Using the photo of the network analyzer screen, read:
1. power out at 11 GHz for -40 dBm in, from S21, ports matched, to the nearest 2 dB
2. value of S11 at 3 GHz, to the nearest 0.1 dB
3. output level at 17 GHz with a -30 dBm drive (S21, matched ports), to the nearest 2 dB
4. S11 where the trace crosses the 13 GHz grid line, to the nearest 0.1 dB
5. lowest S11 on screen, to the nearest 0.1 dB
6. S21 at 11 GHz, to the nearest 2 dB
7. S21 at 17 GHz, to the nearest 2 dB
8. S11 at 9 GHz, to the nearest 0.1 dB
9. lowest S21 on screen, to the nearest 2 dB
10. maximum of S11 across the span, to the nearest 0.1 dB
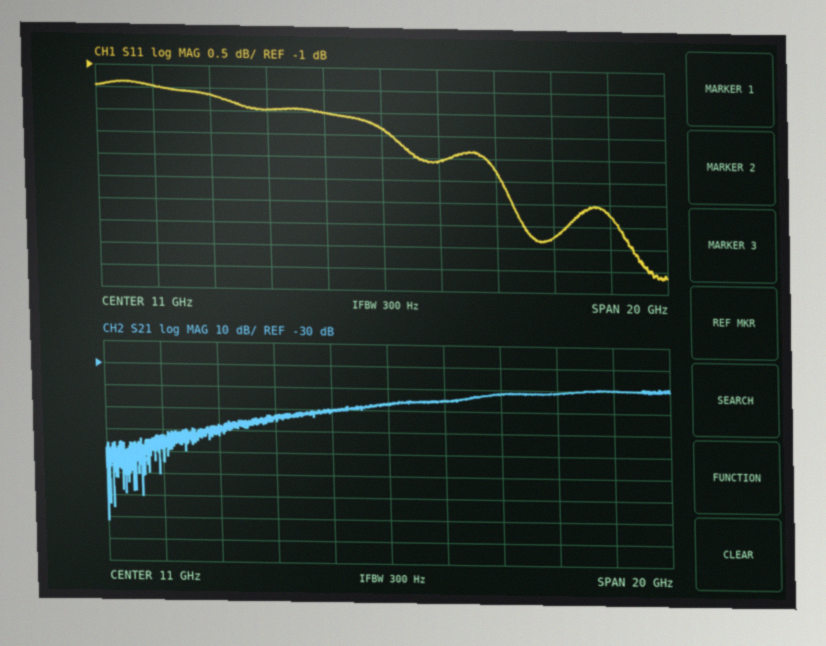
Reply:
-88 dBm
-1.5 dB
-72 dBm
-3.1 dB
-5.7 dB
-48 dB
-42 dB
-2.0 dB
-102 dB
-1.4 dB
